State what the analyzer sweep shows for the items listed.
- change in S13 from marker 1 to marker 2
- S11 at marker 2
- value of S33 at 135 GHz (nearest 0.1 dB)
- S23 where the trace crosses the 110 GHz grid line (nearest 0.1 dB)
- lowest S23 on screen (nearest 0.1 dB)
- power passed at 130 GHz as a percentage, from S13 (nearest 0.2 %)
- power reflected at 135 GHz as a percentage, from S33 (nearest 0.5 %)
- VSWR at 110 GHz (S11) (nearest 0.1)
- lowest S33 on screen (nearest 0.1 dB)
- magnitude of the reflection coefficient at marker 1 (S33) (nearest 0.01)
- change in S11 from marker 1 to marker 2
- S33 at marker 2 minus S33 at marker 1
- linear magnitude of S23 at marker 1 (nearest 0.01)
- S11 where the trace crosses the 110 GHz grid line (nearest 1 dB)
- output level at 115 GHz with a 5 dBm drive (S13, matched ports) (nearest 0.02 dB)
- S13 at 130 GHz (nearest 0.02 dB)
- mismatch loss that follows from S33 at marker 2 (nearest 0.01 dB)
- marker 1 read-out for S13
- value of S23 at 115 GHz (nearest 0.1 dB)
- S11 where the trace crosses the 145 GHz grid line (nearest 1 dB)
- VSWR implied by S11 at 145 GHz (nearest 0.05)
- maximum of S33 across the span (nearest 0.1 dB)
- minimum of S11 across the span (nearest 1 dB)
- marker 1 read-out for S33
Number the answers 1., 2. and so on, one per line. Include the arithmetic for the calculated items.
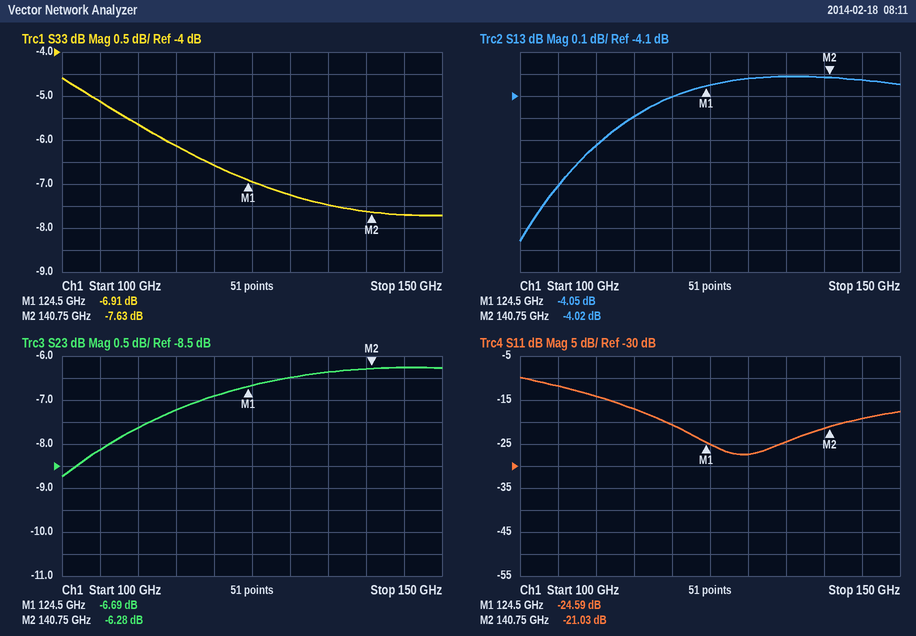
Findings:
1. -4.02 − (-4.05) = 0.03 dB
2. -21.03 dB
3. -7.5 dB
4. -7.6 dB
5. -8.7 dB
6. 10^(-4.02/10) ≈ 39.6 %
7. 10^(-7.5/10) ≈ 17.8 %, so 18.0 % to the nearest 0.5 %
8. |Γ| = 10^(-14/20) = 0.1995; VSWR = (1 + 0.1995)/(1 − 0.1995) ≈ 1.5
9. -7.7 dB
10. 10^(-6.91/20) ≈ 0.45
11. -21.03 − (-24.59) = 3.56 dB
12. -7.63 − (-6.91) = -0.72 dB
13. 10^(-6.69/20) ≈ 0.46
14. -14 dB
15. 5 dBm + (-4.20 dB) = 0.80 dBm
16. -4.02 dB
17. −10 log10(1 − 10^(-7.63/10)) ≈ 0.82 dB
18. -4.05 dB
19. -7.2 dB
20. -19 dB
21. |Γ| = 10^(-19/20) = 0.1122; VSWR = (1 + 0.1122)/(1 − 0.1122) ≈ 1.25
22. -4.6 dB
23. -27 dB
24. -6.91 dB
